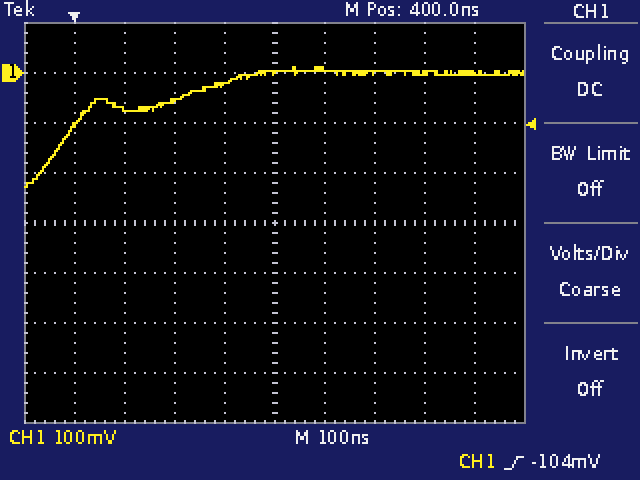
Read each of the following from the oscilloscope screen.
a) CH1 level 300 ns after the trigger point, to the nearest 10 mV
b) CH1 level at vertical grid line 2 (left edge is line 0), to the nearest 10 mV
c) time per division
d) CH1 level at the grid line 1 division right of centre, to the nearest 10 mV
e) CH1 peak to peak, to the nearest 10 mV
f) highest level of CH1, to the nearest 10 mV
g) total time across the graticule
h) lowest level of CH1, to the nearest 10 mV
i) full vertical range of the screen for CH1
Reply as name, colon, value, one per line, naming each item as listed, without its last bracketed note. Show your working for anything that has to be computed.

CH1 level 300 ns after the trigger point, to the nearest 10 mV: -20 mV
CH1 level at vertical grid line 2 (left edge is line 0), to the nearest 10 mV: -70 mV
time per division: 100 ns
CH1 level at the grid line 1 division right of centre, to the nearest 10 mV: 10 mV
CH1 peak to peak, to the nearest 10 mV: 10 mV − (-230 mV) = 240 mV
highest level of CH1, to the nearest 10 mV: 10 mV
total time across the graticule: 1 µs
lowest level of CH1, to the nearest 10 mV: -230 mV
full vertical range of the screen for CH1: 800 mV
